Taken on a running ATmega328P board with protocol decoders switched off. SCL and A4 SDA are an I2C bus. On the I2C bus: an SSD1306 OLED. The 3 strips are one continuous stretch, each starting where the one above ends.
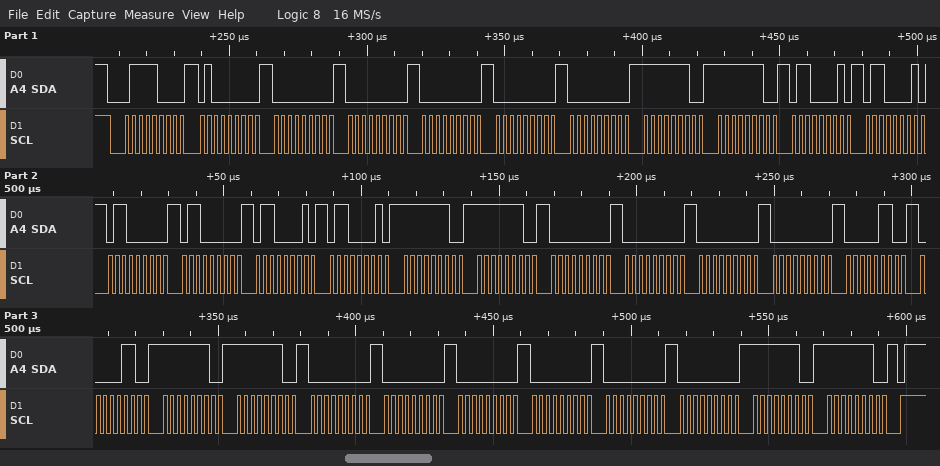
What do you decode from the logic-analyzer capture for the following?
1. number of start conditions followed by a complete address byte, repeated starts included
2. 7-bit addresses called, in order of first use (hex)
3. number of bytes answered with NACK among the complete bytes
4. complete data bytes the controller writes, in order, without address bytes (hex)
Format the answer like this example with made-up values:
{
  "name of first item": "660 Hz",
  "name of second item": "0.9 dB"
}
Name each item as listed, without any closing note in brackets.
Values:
{
  "number of start conditions followed by a complete address byte, repeated starts included": "1",
  "7-bit addresses called, in order of first use": "0x3C",
  "number of bytes answered with NACK among the complete bytes": "0",
  "complete data bytes the controller writes, in order, without address bytes": "40 00 00 00 00 00 FE FE 61 61 60 60 61 61 FE FE 00 00 00 00 06 06 FE FE 00 00 00 00 00 00 FE FE"
}
